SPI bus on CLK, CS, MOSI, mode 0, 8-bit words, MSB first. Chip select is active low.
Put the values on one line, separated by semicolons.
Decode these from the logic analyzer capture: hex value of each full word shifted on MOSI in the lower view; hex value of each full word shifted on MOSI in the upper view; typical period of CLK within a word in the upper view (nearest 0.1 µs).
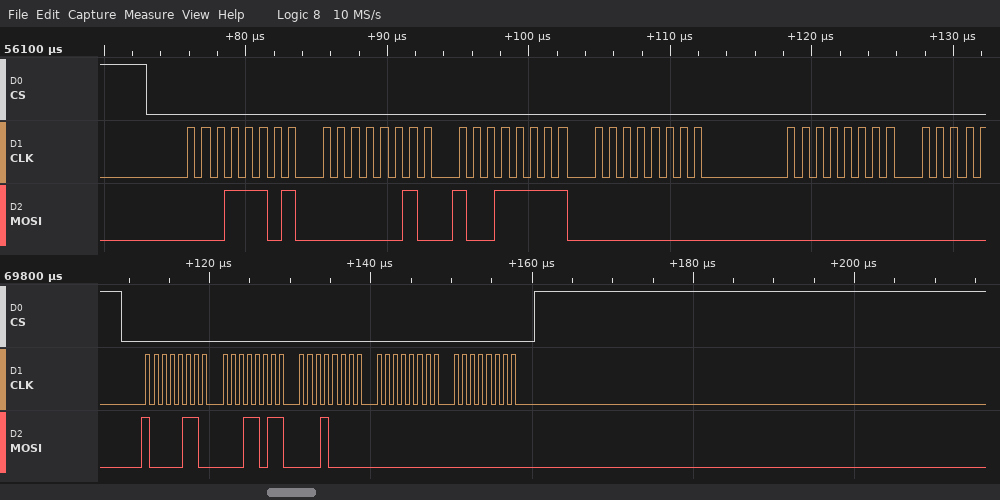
86, 1B, 10, 00, 00; 1D, 02, 9F, 00, 00; 1 µs
